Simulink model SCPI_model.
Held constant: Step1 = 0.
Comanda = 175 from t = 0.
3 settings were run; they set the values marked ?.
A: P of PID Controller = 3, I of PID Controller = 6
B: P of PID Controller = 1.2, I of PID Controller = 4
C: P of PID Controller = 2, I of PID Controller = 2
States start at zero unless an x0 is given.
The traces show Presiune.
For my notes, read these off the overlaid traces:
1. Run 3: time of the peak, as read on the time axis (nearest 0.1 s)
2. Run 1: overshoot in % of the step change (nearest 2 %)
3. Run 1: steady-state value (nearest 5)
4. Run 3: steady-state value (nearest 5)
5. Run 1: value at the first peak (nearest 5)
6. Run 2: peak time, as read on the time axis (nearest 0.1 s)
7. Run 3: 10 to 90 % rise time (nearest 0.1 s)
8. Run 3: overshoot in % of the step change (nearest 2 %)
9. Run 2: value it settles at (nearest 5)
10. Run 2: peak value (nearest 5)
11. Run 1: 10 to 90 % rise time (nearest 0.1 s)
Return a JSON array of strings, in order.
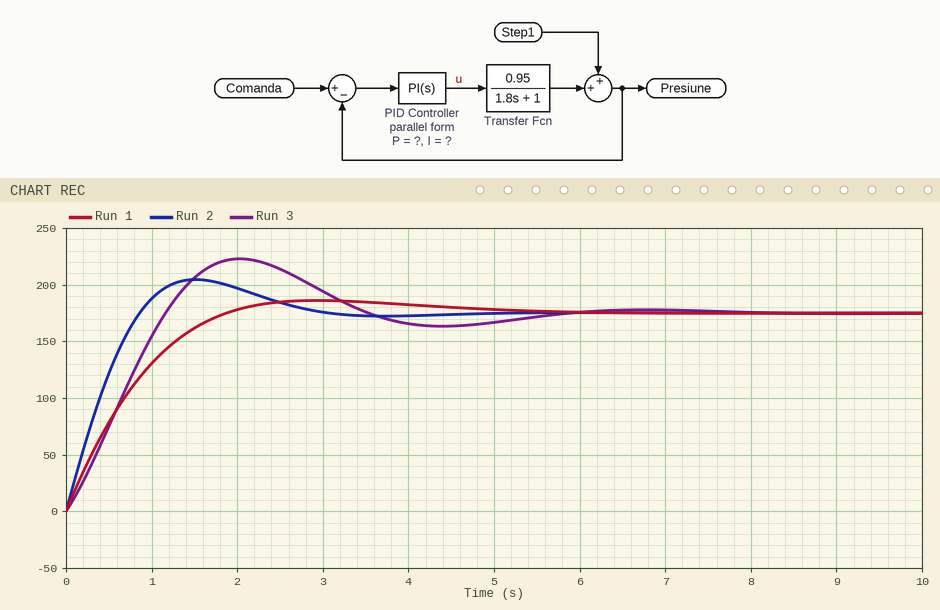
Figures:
["2.0 s", "6 %", "175", "175", "185", "1.5 s", "0.9 s", "28 %", "175", "205", "1.3 s"]
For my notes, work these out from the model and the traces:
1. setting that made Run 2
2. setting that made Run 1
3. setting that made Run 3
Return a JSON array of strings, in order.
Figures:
["A", "C", "B"]
